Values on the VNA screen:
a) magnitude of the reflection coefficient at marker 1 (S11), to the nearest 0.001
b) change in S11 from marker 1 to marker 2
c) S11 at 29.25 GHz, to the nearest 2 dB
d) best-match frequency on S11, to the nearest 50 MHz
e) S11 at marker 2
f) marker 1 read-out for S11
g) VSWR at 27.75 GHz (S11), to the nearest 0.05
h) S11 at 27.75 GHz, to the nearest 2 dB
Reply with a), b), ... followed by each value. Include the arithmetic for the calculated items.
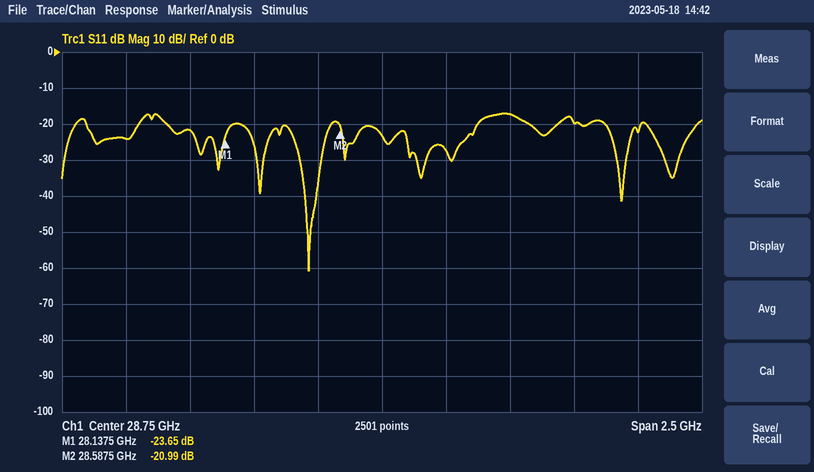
a) 10^(-23.65/20) ≈ 0.066
b) -20.99 − (-23.65) = 2.66 dB
c) -18 dB
d) 28.45 GHz
e) -20.99 dB
f) -23.65 dB
g) |Γ| = 10^(-24/20) = 0.0631; VSWR = (1 + 0.0631)/(1 − 0.0631) ≈ 1.13, so 1.15 to the nearest 0.05
h) -24 dB
